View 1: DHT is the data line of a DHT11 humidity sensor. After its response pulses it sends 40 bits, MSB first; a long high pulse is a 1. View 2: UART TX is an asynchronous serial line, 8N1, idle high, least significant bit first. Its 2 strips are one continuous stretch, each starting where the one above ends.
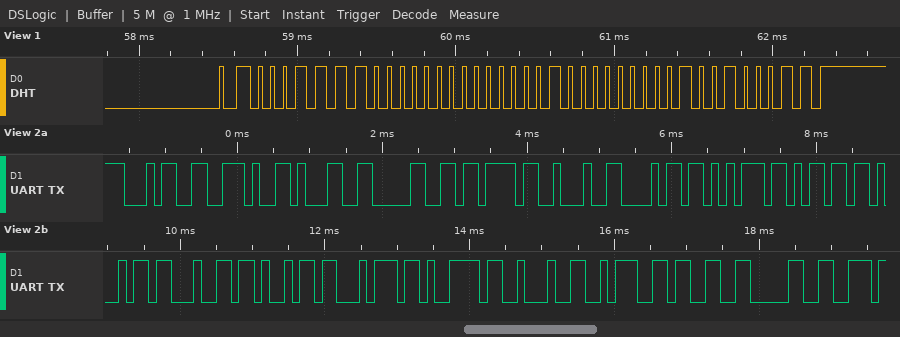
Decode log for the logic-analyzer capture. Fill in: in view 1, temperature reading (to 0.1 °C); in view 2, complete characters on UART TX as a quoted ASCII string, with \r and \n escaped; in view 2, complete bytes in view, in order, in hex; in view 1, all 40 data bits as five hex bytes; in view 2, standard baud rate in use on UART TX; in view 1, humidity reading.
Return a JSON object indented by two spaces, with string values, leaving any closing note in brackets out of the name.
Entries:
{
  "in view 1, temperature reading": "4.1 °C",
  "in view 2, complete characters on UART TX as a quoted ASCII string, with \\r and \\n escaped": "\"4.10{\\\"humidity\\\":30\"",
  "in view 2, complete bytes in view, in order, in hex": "34 2E 31 30 7B 22 68 75 6D 69 64 69 74 79 22 3A 33 30",
  "in view 1, all 40 data bits as five hex bytes": "1E 00 04 01 23",
  "in view 2, standard baud rate in use on UART TX": "9600 baud",
  "in view 1, humidity reading": "30 %"
}
